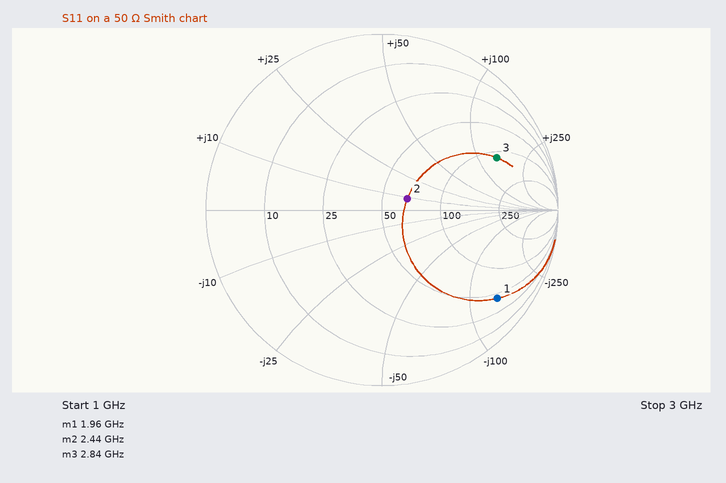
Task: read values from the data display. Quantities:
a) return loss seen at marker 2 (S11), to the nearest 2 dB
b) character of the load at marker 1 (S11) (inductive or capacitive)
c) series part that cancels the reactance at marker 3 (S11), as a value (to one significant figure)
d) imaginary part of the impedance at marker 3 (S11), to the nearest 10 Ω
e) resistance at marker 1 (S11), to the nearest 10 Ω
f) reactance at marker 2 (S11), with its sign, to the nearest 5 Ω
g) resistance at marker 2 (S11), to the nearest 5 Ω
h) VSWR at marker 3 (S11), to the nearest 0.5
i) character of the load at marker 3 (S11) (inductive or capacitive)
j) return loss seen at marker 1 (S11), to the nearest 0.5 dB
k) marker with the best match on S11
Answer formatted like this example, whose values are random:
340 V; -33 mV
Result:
16 dB; capacitive; 400 fF; +140 Ω; 40 Ω; +10 Ω; 65 Ω; 6.0; inductive; 1.5 dB; marker 2
